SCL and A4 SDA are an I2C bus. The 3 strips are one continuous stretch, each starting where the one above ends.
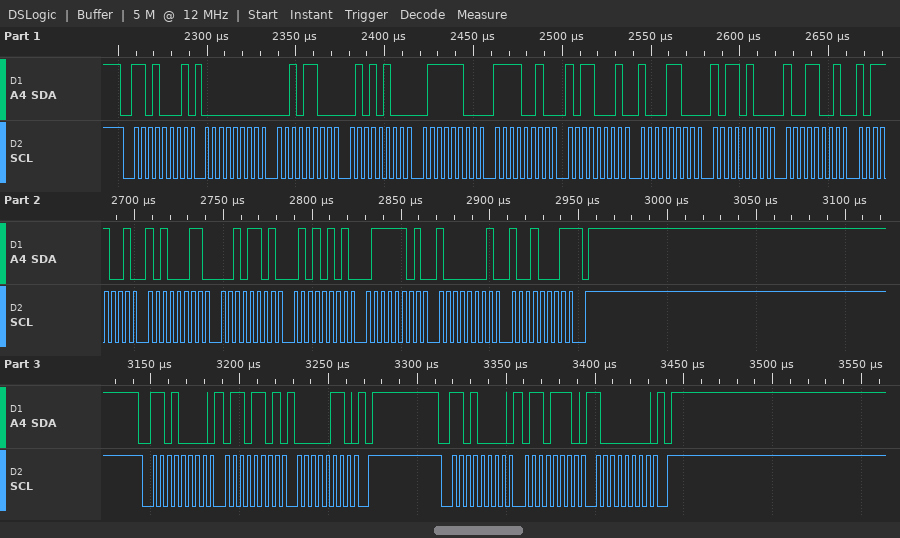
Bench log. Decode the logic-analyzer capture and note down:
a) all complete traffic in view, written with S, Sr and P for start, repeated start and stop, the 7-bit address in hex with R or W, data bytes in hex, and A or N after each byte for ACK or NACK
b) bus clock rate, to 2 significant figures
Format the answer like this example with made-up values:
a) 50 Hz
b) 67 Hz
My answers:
a) S 68R A 00 A 2C A 54 A 7C A F2 A B1 A 8C A B4 A 99 A B9 A A3 A 2D A 55 A 7D A 81 A 91 N P S 68W A 6D A 06 A P S 68W A 6E A 80 A P
b) 250 kHz
